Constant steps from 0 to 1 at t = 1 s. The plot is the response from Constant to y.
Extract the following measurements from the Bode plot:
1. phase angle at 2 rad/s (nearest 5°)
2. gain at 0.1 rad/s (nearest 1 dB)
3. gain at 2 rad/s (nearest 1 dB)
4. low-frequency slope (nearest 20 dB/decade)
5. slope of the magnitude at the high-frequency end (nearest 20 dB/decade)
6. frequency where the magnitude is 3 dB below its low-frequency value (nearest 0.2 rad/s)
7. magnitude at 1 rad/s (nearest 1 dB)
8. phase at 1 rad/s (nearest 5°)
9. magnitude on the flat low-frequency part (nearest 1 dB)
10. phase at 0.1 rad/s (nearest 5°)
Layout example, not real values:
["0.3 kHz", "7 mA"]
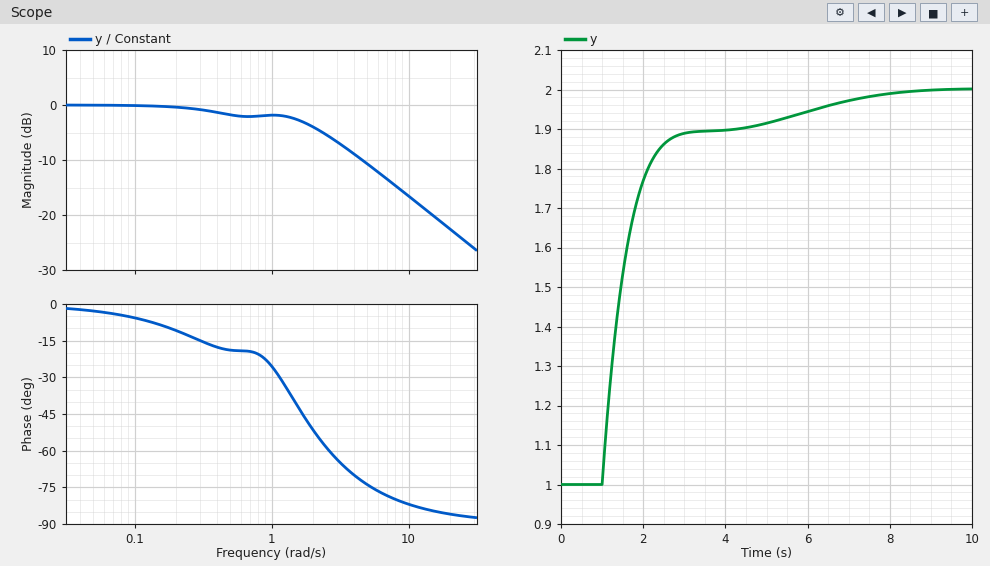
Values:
["-50°", "0 dB", "-4 dB", "0 dB/decade", "-20 dB/decade", "1.6 rad/s", "-2 dB", "-25°", "0 dB", "-5°"]
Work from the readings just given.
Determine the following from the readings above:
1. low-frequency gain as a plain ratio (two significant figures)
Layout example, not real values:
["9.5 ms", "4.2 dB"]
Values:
["1.0"]
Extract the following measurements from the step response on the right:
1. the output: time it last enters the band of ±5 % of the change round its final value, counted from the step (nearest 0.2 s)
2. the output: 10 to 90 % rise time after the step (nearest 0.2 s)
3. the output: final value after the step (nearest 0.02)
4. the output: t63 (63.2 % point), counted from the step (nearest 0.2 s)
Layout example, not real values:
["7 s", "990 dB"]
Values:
["5.2 s", "3.2 s", "2.00", "0.6 s"]
